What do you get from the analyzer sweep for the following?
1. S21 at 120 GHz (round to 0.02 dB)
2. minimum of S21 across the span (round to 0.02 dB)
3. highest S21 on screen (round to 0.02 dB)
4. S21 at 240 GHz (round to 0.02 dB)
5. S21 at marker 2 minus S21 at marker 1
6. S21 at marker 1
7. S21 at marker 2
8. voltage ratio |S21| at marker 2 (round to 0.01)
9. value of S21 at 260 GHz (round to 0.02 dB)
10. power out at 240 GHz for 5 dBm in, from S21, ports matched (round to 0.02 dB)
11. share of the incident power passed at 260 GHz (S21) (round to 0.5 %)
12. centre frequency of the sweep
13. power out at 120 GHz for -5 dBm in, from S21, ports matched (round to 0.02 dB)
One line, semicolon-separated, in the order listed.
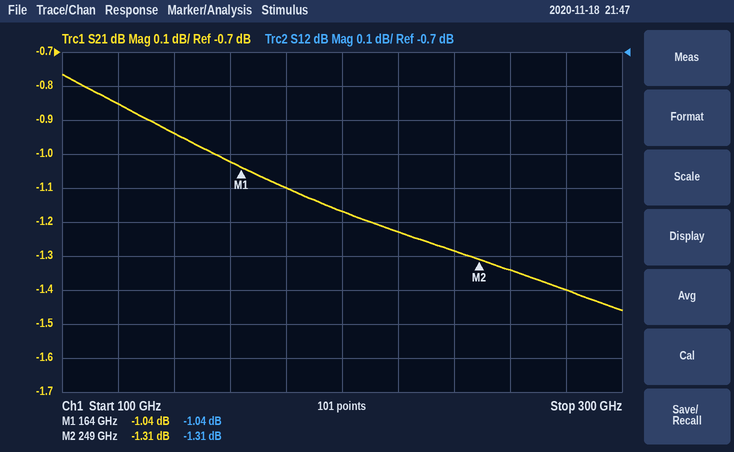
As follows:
-0.86 dB; -1.46 dB; -0.76 dB; -1.28 dB; -0.27 dB; -1.04 dB; -1.31 dB; 0.86; -1.34 dB; 3.72 dBm; 73.5 %; 200 GHz; -5.86 dBm
